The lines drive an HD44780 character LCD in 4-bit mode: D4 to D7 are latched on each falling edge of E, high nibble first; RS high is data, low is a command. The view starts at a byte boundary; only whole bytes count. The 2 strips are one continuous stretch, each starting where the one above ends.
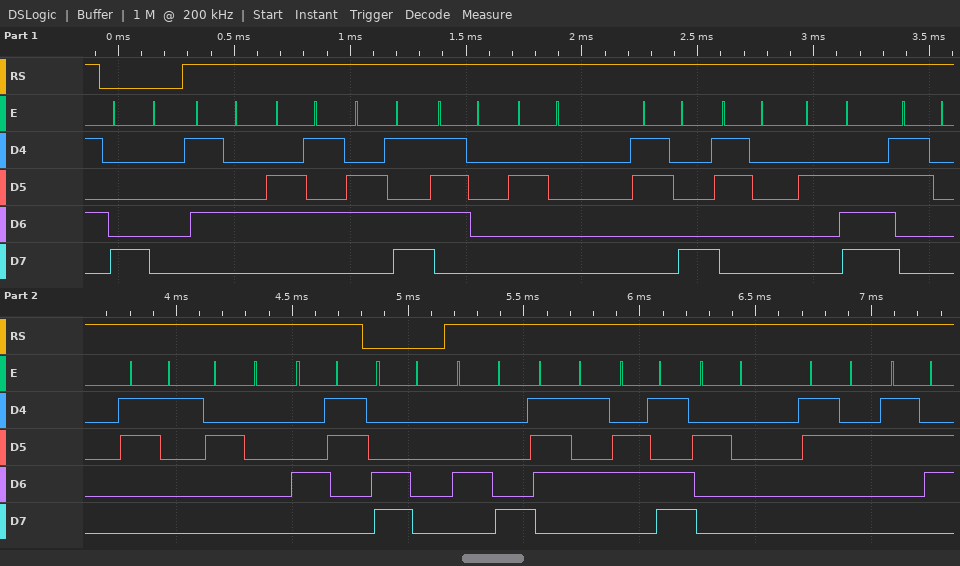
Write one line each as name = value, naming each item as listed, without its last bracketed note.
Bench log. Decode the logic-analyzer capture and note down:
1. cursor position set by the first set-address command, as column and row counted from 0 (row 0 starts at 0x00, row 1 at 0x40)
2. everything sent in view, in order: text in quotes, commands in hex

cursor position set by the first set-address command, as column and row counted from 0 = column 0, row 0
everything sent in view, in order: text in quotes, commands in hex = 0x80 "Temp 80.01 C" 0xC0 "Hum 26"
